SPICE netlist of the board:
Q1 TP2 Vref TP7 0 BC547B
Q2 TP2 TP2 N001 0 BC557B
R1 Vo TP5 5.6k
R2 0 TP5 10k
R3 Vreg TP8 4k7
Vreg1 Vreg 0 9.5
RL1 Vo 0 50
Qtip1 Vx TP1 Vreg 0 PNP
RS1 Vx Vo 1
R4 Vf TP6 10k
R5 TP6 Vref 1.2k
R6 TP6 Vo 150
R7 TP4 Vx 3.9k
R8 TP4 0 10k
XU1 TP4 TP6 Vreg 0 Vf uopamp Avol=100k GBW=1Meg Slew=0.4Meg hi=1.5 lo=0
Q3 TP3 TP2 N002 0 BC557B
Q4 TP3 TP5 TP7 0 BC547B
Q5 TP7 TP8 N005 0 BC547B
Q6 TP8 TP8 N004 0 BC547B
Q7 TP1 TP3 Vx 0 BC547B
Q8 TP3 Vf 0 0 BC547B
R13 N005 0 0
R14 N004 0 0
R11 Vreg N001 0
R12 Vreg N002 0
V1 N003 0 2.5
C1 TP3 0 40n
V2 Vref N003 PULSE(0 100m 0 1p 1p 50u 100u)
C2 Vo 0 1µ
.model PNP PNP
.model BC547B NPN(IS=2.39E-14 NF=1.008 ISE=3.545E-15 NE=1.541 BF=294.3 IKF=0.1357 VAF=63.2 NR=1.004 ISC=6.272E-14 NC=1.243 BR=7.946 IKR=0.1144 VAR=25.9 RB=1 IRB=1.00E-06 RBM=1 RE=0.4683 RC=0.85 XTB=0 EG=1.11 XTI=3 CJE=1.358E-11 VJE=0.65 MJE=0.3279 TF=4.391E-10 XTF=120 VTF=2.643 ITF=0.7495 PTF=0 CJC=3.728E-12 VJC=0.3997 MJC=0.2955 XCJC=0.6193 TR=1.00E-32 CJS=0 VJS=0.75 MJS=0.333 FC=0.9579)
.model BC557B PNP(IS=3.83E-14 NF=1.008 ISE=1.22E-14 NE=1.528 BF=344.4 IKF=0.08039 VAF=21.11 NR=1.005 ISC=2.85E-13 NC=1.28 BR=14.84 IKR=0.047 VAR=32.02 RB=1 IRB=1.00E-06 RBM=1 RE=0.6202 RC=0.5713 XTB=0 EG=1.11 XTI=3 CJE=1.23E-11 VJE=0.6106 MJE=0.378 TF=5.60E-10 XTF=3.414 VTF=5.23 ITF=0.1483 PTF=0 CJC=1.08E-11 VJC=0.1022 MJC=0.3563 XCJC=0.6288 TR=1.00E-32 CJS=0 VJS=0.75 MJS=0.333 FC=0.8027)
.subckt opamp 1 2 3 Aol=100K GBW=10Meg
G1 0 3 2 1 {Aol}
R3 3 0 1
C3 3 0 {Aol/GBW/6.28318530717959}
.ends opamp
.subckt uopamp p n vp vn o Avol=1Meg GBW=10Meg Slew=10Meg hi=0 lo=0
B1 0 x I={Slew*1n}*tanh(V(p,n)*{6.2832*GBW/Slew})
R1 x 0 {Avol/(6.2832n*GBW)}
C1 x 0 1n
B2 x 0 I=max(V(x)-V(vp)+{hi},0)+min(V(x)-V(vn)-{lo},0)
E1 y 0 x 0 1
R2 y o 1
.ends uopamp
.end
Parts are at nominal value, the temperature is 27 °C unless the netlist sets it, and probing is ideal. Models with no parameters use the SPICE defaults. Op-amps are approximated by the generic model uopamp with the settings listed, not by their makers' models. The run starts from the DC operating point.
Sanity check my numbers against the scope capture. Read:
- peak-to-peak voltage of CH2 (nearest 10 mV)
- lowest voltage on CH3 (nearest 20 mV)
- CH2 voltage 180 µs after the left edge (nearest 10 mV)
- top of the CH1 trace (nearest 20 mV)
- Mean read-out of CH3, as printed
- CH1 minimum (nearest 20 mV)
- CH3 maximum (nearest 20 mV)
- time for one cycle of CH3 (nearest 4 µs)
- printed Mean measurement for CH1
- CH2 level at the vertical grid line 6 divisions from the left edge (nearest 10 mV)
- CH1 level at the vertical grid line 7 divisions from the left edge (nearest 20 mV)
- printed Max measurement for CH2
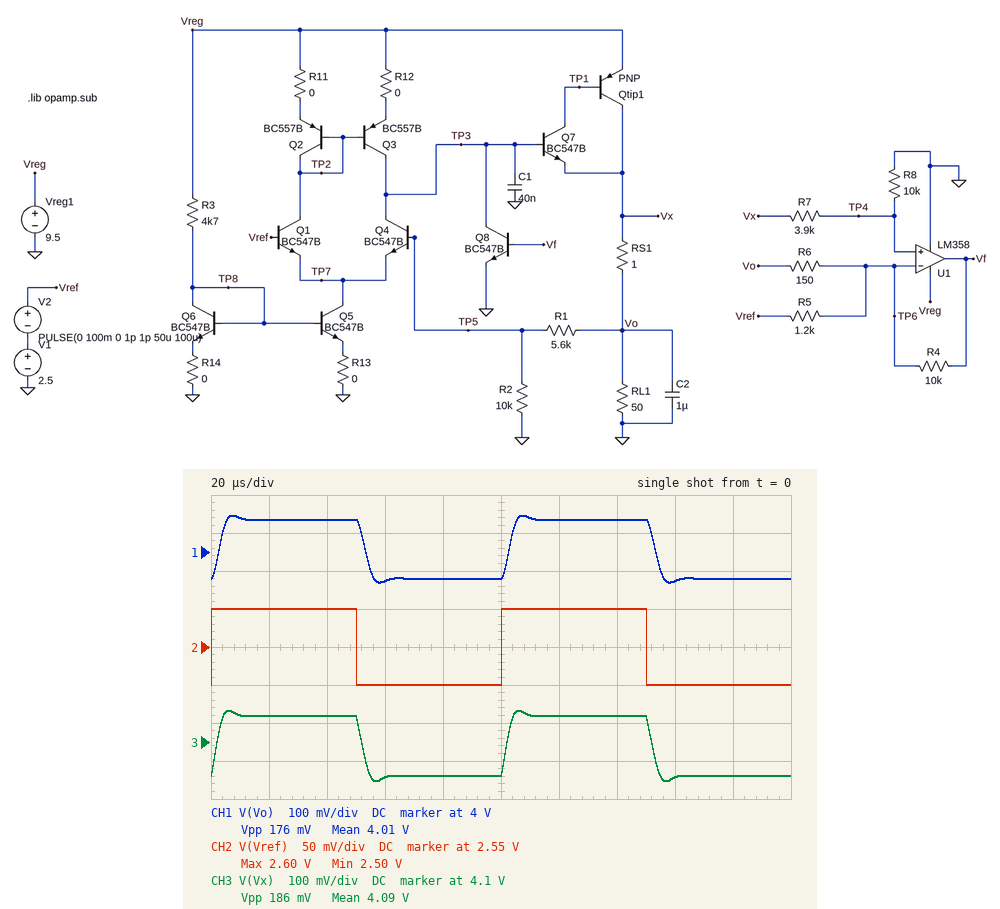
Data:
100 mV
4.00 V
2.50 V
4.10 V
4.09 V
3.92 V
4.18 V
100 µs
4.01 V
2.60 V
4.08 V
2.60 V
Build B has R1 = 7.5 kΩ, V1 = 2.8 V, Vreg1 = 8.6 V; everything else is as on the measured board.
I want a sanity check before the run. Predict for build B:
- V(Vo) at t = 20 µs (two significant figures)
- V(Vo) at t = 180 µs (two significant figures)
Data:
5.1 V
4.9 V
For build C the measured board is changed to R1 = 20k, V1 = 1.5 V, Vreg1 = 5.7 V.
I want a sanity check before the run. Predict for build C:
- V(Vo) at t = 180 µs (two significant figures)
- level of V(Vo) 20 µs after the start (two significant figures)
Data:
4.5 V
4.7 V
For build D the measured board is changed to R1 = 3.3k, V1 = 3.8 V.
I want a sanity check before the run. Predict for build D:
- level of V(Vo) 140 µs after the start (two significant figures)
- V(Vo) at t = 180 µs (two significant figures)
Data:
5.2 V
5.1 V
